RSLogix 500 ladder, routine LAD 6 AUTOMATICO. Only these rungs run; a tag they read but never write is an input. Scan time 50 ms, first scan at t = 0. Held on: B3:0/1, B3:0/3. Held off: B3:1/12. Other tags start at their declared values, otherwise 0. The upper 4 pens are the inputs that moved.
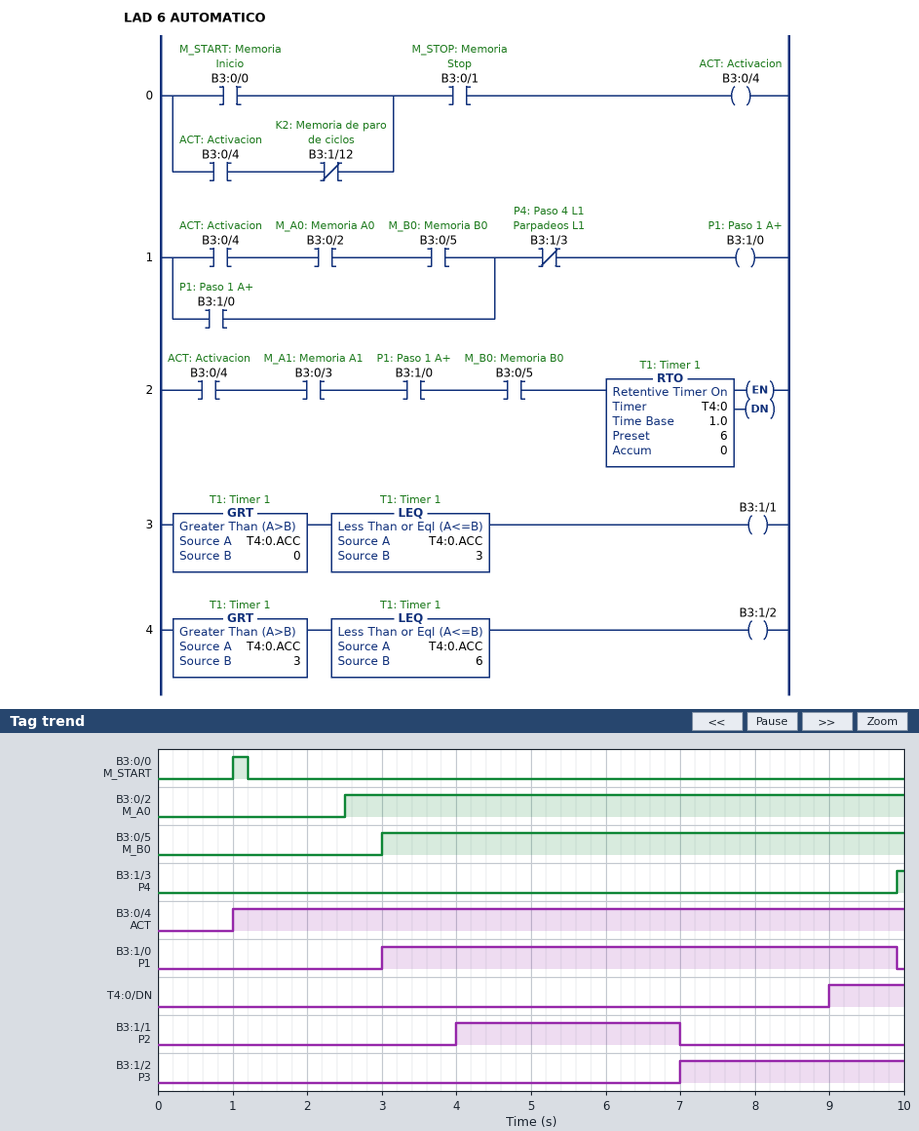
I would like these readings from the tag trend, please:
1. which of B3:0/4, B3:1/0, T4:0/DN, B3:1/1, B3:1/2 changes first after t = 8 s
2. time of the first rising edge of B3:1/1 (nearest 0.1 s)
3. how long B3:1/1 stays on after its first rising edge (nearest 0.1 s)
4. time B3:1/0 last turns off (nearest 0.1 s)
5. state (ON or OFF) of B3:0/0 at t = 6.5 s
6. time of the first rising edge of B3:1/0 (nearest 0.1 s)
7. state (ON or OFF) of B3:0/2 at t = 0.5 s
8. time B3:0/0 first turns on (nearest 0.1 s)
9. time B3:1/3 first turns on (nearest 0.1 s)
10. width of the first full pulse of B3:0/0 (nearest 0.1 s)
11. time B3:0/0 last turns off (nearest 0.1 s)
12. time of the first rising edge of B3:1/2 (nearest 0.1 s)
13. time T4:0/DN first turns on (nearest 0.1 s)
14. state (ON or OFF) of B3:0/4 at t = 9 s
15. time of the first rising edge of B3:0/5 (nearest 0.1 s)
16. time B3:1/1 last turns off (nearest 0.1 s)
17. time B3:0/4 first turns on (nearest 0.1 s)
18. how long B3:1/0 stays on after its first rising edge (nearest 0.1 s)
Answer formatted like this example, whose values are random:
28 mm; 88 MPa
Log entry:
T4:0/DN; 4.0 s; 3.0 s; 9.9 s; OFF; 3.0 s; OFF; 1.0 s; 9.9 s; 0.2 s; 1.2 s; 7.0 s; 9.0 s; ON; 3.0 s; 7.0 s; 1.0 s; 6.9 s
